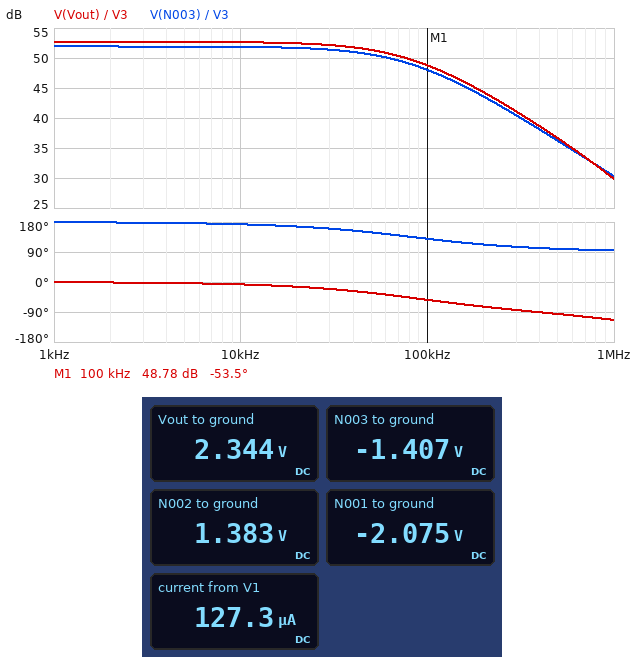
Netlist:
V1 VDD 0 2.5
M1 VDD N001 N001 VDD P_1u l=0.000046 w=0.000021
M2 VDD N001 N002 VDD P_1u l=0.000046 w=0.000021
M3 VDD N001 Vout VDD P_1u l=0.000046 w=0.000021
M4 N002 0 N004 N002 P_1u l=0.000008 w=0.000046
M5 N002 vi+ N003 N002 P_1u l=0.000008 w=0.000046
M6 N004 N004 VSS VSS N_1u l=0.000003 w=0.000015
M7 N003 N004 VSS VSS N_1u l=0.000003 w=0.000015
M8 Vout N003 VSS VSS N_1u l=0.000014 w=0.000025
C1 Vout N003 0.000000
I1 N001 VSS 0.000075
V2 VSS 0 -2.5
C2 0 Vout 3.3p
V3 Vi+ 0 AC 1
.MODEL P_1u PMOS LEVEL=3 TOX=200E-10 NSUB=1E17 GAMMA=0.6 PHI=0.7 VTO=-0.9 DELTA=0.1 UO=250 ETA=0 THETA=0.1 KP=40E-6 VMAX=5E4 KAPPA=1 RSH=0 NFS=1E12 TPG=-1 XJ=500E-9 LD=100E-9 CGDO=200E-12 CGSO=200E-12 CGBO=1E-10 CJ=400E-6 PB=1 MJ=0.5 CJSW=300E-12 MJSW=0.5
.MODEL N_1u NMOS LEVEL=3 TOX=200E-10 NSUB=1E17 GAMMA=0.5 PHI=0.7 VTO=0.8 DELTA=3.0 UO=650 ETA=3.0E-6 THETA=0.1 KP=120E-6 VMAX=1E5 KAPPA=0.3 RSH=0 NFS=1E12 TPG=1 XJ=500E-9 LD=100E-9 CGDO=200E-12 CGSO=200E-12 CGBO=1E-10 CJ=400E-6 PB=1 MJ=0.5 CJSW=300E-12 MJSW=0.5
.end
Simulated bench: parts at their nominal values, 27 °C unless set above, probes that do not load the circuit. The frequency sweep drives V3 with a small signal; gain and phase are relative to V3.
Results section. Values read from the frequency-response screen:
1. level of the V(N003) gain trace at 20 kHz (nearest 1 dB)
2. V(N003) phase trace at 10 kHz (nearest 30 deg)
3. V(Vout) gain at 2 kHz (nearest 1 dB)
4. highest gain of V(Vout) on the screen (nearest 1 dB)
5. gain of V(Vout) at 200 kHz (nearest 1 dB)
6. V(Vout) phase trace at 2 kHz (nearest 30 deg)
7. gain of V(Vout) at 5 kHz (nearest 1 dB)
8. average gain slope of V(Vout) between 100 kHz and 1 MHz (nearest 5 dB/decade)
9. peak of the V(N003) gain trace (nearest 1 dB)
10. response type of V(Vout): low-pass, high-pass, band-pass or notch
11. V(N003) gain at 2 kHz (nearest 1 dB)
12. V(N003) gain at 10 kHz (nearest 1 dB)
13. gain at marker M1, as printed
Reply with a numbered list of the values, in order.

1. 52 dB
2. 180 deg
3. 53 dB
4. 53 dB
5. 44 dB
6. 0 deg
7. 53 dB
8. -20 dB/decade
9. 52 dB
10. low-pass
11. 52 dB
12. 52 dB
13. 48.78 dB
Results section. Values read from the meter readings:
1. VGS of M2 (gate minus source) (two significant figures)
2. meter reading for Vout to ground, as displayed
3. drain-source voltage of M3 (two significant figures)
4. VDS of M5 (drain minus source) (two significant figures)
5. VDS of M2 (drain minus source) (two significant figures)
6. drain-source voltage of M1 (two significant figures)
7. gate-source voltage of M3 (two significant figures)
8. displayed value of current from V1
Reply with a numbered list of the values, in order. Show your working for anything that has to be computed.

1. -2.075 V - 1.383 V = -3.5 V
2. 2.344 V
3. 2.5 V - 2.344 V = 160 mV
4. 1.383 V - (-1.407 V) = 2.8 V
5. 2.5 V - 1.383 V = 1.1 V
6. 2.5 V - (-2.075 V) = 4.6 V
7. -2.075 V - 2.344 V = -4.4 V
8. 127.3 µA
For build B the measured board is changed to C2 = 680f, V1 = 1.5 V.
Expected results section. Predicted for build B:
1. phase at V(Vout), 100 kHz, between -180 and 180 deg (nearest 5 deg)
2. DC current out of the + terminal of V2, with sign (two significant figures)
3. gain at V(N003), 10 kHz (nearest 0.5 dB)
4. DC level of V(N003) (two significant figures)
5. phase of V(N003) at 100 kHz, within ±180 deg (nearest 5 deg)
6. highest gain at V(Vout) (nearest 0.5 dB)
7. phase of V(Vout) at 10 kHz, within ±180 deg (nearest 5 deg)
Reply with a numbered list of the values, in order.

1. -80 deg
2. -93 µA
3. 59.0 dB
4. -1.5 V
5. 100 deg
6. 55.5 dB
7. -25 deg
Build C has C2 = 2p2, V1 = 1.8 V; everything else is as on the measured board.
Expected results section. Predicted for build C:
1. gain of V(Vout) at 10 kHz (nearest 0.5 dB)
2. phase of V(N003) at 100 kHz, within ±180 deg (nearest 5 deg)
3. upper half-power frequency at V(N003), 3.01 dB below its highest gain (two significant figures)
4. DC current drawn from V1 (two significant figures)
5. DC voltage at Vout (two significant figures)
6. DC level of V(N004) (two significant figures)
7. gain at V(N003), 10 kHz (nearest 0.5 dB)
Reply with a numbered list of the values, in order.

1. 54.0 dB
2. 110 deg
3. 38 kHz
4. 100 µA
5. 1.7 V
6. -1.5 V
7. 56.0 dB
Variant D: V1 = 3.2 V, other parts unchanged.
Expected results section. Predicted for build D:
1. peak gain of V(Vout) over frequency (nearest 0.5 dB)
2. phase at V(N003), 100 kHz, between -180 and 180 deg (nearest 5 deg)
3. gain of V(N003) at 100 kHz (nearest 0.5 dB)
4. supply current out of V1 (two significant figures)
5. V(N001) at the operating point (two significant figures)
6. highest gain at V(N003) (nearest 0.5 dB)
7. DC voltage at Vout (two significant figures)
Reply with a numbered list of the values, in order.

1. 52.0 dB
2. 140 deg
3. 47.5 dB
4. 150 µA
5. -1.4 V
6. 50.0 dB
7. 3.0 V
